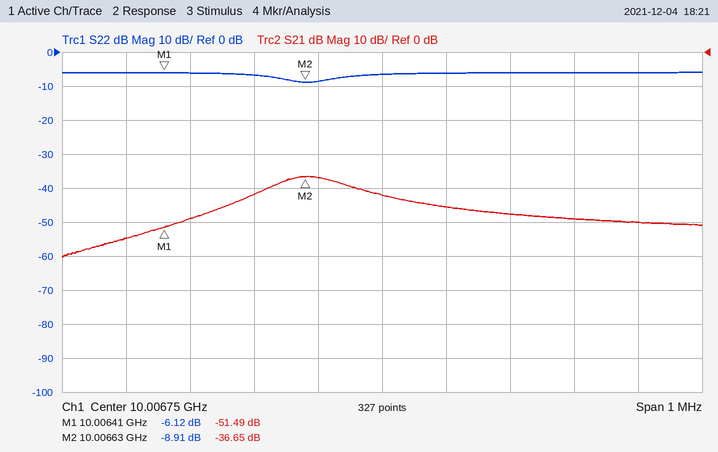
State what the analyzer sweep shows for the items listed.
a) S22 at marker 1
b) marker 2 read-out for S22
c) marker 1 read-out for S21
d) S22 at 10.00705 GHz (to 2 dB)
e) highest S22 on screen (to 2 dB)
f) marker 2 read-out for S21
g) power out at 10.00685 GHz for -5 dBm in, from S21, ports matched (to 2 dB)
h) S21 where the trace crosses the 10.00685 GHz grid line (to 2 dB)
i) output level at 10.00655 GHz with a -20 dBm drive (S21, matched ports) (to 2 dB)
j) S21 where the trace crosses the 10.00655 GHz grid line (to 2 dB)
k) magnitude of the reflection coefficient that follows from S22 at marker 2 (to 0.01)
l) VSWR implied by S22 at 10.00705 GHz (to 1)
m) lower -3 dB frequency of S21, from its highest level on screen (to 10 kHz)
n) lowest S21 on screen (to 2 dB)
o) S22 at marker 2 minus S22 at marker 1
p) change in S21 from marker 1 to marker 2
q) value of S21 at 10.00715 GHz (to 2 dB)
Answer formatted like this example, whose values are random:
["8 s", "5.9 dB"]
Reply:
["-6.12 dB", "-8.91 dB", "-51.49 dB", "-6 dB", "-6 dB", "-36.65 dB", "-50 dBm", "-46 dB", "-62 dBm", "-42 dB", "0.36", "3", "10.00658 GHz", "-60 dB", "-2.79 dB", "14.84 dB", "-50 dB"]
